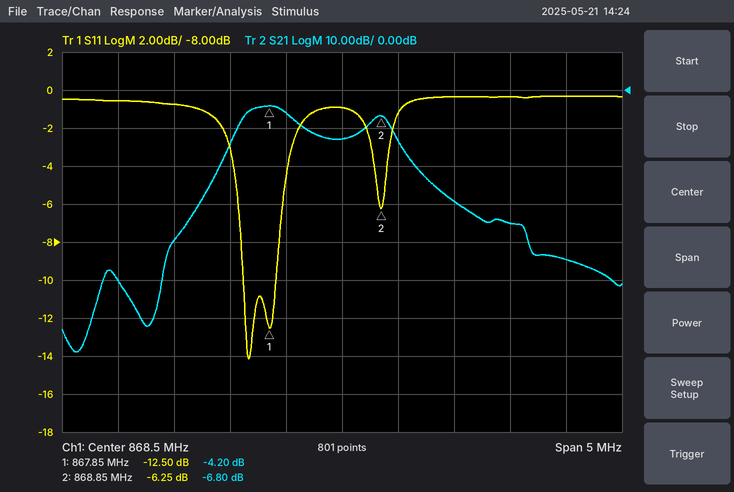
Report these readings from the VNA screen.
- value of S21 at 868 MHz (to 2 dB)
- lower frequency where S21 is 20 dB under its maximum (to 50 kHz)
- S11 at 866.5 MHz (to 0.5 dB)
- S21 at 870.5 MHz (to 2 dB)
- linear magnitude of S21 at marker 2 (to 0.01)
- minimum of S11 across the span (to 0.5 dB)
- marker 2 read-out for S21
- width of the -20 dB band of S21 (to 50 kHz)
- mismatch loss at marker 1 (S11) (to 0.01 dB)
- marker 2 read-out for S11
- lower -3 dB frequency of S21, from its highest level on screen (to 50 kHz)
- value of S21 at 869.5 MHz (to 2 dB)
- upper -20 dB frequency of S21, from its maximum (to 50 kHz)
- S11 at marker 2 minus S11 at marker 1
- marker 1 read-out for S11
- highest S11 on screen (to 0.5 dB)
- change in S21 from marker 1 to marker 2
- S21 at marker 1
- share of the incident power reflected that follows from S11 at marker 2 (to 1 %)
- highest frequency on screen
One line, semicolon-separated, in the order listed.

-6 dB; 867.35 MHz; -0.5 dB; -44 dB; 0.46; -14.0 dB; -6.80 dB; 1.95 MHz; 0.25 dB; -6.25 dB; 867.60 MHz; -30 dB; 869.30 MHz; 6.25 dB; -12.50 dB; -0.5 dB; -2.60 dB; -4.20 dB; 24 %; 871 MHz
